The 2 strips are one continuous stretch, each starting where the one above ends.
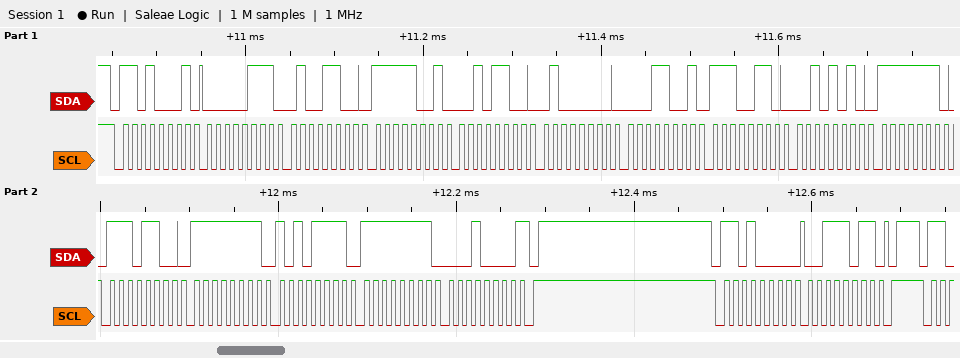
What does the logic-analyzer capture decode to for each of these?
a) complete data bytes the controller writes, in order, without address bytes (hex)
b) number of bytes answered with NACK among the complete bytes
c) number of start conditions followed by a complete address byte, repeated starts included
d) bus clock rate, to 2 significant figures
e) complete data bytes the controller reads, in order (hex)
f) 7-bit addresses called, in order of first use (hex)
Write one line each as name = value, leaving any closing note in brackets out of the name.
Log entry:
complete data bytes the controller writes, in order, without address bytes = 3B
number of bytes answered with NACK among the complete bytes = 1
number of start conditions followed by a complete address byte, repeated starts included = 2
bus clock rate, to 2 significant figures = 100 kHz
complete data bytes the controller reads, in order = 07 4C F9 2C 40 19 E6 2A FE EC FF AF FF 10
7-bit addresses called, in order of first use = 0x68
